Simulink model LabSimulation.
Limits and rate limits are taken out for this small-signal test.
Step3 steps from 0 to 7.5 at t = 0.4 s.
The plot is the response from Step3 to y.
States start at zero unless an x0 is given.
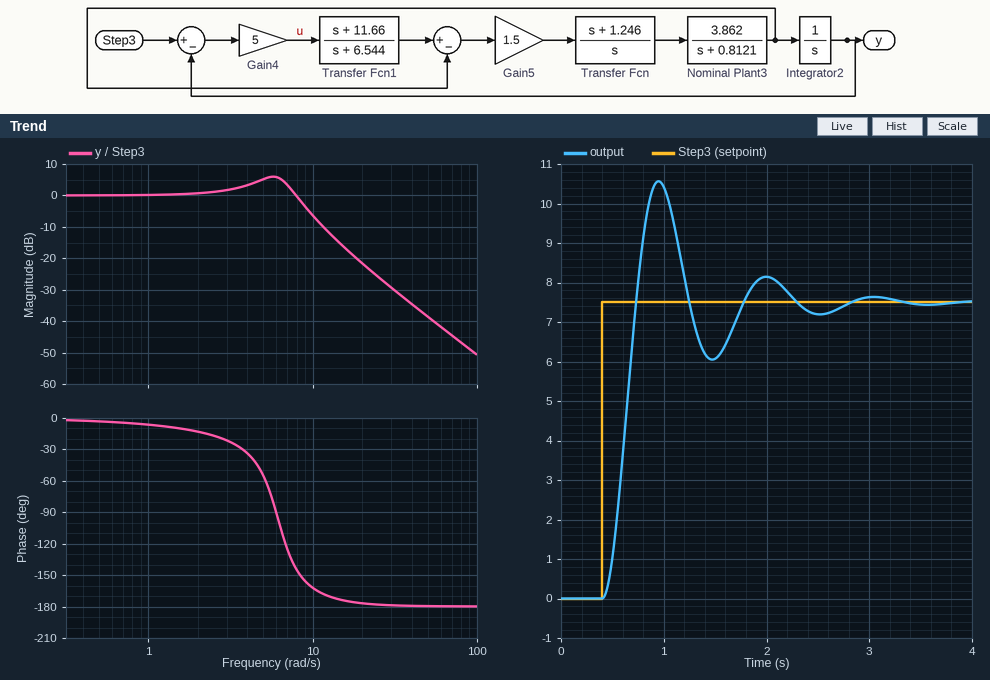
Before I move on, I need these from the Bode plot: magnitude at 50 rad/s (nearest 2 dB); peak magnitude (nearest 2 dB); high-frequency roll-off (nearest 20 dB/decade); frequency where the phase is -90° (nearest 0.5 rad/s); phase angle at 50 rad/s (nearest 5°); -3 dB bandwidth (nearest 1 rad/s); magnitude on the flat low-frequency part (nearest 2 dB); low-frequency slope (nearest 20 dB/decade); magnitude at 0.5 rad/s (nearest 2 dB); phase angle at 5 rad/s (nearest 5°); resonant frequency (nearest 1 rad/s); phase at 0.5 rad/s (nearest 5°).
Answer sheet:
-38 dB
6 dB
-40 dB/decade
6.0 rad/s
-180°
9 rad/s
0 dB
0 dB/decade
0 dB
-55°
6 rad/s
-5°
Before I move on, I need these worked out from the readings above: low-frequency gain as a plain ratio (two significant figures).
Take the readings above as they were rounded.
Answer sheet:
1.0
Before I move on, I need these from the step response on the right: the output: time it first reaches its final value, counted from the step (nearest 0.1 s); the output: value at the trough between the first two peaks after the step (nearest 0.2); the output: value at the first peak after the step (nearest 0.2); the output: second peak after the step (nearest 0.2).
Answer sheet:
0.3 s
6.0
10.6
8.2
